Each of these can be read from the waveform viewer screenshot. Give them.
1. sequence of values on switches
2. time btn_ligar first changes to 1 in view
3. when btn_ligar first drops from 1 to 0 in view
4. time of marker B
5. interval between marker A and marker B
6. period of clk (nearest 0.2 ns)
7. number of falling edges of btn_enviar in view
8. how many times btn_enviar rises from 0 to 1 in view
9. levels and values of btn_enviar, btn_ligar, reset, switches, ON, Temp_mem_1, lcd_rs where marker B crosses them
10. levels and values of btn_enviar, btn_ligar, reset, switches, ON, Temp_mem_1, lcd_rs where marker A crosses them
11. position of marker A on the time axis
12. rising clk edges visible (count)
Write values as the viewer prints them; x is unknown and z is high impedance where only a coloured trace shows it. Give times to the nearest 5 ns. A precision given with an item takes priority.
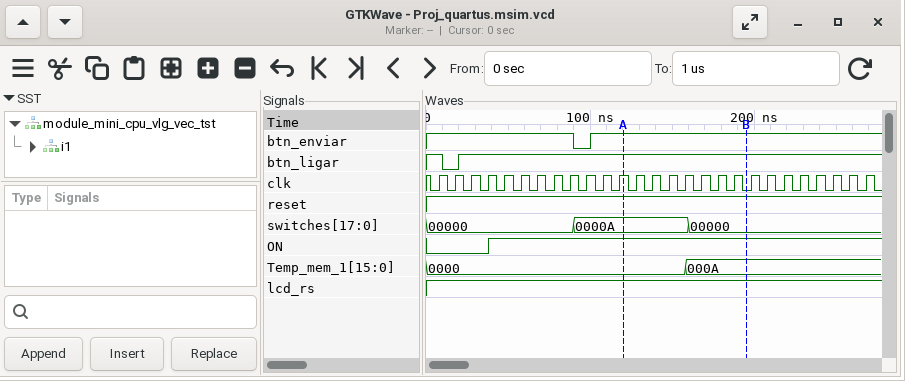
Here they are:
00000, 0000A, 00000
20 ns
10 ns
195 ns
75 ns
10 ns
1
1
btn_enviar=1, btn_ligar=1, reset=1, switches=00000, ON=1, Temp_mem_1=000A, lcd_rs=1
btn_enviar=1, btn_ligar=1, reset=1, switches=0000A, ON=1, Temp_mem_1=0000, lcd_rs=1
120 ns
27
